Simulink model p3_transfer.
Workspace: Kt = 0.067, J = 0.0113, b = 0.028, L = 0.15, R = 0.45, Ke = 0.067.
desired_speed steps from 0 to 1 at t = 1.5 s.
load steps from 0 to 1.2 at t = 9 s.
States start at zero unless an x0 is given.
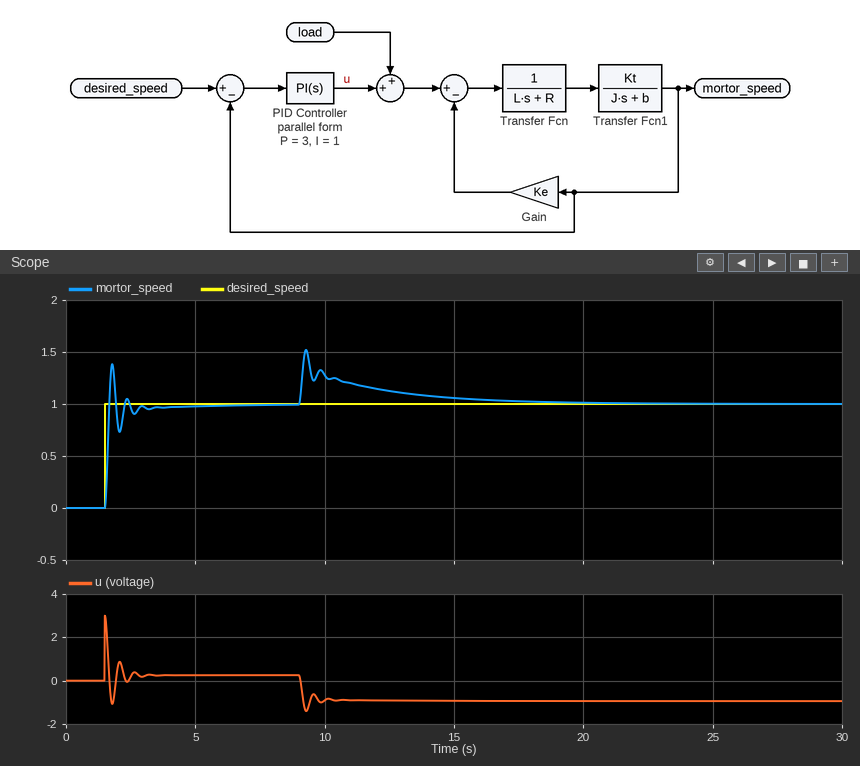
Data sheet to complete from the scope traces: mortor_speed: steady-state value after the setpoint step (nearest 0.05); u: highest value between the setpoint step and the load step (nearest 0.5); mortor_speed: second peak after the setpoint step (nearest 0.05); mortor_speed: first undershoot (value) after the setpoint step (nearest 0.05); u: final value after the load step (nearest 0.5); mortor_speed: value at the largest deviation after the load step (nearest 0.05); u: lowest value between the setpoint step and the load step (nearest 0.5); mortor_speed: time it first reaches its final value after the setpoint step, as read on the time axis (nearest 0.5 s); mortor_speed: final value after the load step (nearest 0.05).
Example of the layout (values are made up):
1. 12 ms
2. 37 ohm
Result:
1. 1.00
2. 3.0
3. 1.05
4. 0.75
5. -1.0
6. 1.50
7. -1.0
8. 1.5 s
9. 1.00
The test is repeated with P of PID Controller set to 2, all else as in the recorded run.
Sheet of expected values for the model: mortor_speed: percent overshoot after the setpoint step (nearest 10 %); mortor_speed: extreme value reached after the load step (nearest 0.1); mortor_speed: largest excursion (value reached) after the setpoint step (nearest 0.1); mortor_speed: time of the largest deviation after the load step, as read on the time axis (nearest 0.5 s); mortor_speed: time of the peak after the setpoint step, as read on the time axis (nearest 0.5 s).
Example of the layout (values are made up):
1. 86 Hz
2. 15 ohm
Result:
1. 30 %
2. 1.7
3. 1.3
4. 9.5 s
5. 2.0 s
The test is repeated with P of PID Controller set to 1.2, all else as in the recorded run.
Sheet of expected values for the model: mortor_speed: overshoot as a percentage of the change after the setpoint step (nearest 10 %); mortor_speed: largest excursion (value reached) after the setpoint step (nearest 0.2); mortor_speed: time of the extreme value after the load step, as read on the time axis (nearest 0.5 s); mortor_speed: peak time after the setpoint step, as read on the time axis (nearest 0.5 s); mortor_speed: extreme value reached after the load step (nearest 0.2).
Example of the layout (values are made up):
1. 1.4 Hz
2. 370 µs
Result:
1. 20 %
2. 1.2
3. 9.5 s
4. 2.0 s
5. 2.0
